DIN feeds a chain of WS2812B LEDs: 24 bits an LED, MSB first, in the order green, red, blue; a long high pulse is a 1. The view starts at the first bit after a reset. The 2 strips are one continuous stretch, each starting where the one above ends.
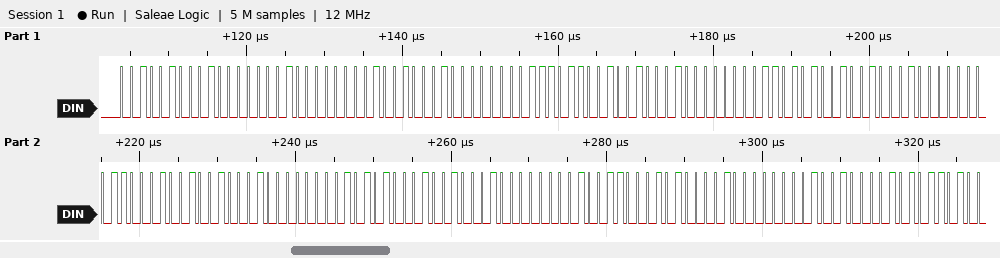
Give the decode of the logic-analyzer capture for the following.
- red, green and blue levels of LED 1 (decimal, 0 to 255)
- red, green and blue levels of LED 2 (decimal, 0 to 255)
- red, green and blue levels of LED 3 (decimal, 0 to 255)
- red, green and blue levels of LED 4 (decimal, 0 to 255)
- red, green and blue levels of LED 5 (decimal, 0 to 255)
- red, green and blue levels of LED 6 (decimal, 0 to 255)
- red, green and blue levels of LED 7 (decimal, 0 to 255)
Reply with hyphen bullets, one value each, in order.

- 64, 36, 64
- 64, 36, 59
- 64, 36, 53
- 64, 36, 49
- 64, 36, 42
- 64, 36, 38
- 64, 40, 36
